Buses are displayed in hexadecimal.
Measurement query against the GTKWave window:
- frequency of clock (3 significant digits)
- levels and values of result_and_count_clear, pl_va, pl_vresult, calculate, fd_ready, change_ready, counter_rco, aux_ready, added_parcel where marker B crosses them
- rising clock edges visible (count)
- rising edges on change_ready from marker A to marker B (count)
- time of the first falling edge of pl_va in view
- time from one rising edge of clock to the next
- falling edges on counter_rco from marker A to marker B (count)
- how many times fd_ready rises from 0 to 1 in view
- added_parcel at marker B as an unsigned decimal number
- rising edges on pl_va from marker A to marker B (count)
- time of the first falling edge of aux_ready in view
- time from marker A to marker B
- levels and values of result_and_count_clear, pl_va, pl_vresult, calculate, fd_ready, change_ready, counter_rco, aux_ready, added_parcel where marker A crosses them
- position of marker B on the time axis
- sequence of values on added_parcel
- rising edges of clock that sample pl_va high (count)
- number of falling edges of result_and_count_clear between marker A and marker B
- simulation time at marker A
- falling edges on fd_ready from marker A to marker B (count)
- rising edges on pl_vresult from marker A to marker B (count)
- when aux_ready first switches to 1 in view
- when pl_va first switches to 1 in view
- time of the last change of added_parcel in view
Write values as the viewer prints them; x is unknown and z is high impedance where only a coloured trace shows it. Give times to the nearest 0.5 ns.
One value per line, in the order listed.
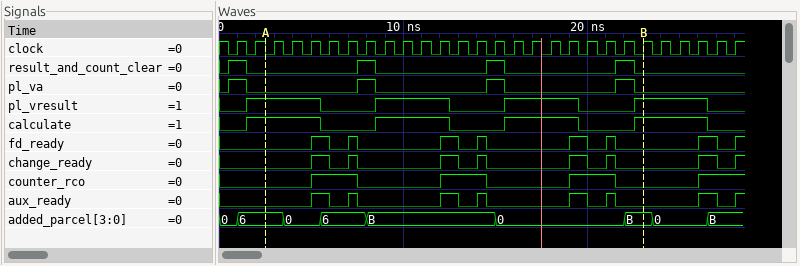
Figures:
1.00 GHz
result_and_count_clear=0, pl_va=0, pl_vresult=1, calculate=1, fd_ready=0, change_ready=0, counter_rco=0, aux_ready=0, added_parcel=B
28
6
1.5 ns
1 ns
3
8
11
3
6 ns
20.5 ns
result_and_count_clear=0, pl_va=0, pl_vresult=1, calculate=1, fd_ready=0, change_ready=0, counter_rco=0, aux_ready=0, added_parcel=6
23 ns
0, 6, 0, 6, B, 0, B, 0, B
4
3
2.5 ns
6
3
5 ns
0.5 ns
26.5 ns
